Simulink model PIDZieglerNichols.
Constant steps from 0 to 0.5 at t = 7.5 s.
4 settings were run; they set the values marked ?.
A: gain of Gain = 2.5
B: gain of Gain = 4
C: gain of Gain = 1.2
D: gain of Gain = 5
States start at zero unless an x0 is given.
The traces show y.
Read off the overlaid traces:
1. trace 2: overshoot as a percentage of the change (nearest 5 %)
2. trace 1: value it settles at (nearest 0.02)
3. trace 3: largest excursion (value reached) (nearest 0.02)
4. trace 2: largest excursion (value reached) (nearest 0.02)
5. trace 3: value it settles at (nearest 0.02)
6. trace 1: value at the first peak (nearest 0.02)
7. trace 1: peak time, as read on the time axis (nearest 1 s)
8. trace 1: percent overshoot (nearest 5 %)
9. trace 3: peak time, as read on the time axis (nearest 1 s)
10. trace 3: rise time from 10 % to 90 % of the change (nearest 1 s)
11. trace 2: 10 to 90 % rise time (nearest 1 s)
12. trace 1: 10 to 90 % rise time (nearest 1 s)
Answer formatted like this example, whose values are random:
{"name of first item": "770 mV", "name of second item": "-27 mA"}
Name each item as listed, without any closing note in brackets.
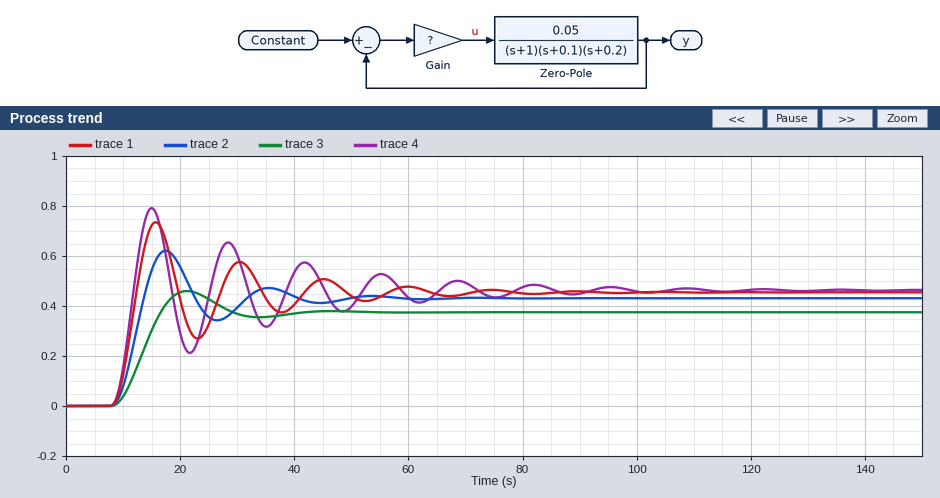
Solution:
{"trace 2: overshoot as a percentage of the change": "45 %", "trace 1: value it settles at": "0.46", "trace 3: largest excursion (value reached)": "0.46", "trace 2: largest excursion (value reached)": "0.62", "trace 3: value it settles at": "0.38", "trace 1: value at the first peak": "0.74", "trace 1: peak time, as read on the time axis": "16 s", "trace 1: percent overshoot": "60 %", "trace 3: peak time, as read on the time axis": "21 s", "trace 3: rise time from 10 % to 90 % of the change": "6 s", "trace 2: 10 to 90 % rise time": "4 s", "trace 1: 10 to 90 % rise time": "3 s"}
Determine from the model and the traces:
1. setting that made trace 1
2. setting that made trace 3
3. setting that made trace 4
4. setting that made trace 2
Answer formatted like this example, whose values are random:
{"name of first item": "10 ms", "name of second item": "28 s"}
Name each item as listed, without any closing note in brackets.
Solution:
{"setting that made trace 1": "B", "setting that made trace 3": "C", "setting that made trace 4": "D", "setting that made trace 2": "A"}
